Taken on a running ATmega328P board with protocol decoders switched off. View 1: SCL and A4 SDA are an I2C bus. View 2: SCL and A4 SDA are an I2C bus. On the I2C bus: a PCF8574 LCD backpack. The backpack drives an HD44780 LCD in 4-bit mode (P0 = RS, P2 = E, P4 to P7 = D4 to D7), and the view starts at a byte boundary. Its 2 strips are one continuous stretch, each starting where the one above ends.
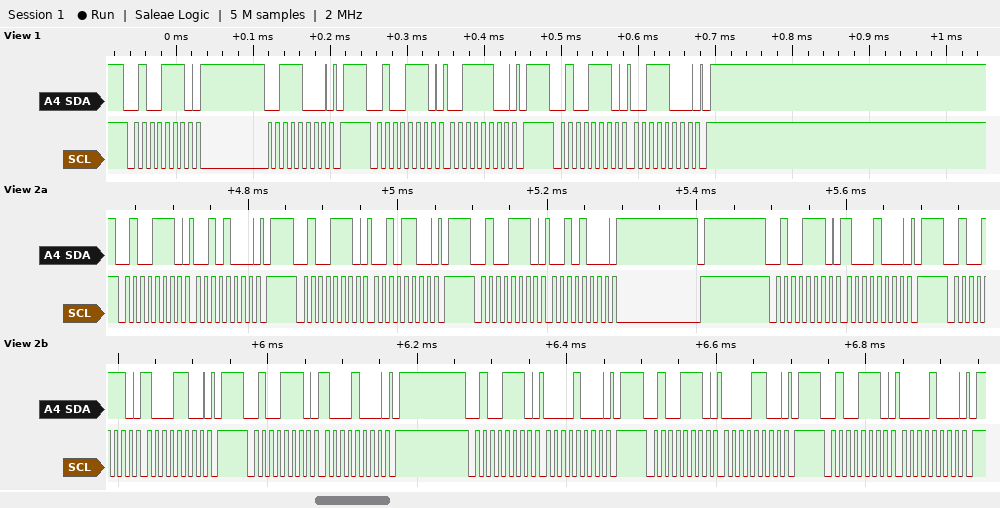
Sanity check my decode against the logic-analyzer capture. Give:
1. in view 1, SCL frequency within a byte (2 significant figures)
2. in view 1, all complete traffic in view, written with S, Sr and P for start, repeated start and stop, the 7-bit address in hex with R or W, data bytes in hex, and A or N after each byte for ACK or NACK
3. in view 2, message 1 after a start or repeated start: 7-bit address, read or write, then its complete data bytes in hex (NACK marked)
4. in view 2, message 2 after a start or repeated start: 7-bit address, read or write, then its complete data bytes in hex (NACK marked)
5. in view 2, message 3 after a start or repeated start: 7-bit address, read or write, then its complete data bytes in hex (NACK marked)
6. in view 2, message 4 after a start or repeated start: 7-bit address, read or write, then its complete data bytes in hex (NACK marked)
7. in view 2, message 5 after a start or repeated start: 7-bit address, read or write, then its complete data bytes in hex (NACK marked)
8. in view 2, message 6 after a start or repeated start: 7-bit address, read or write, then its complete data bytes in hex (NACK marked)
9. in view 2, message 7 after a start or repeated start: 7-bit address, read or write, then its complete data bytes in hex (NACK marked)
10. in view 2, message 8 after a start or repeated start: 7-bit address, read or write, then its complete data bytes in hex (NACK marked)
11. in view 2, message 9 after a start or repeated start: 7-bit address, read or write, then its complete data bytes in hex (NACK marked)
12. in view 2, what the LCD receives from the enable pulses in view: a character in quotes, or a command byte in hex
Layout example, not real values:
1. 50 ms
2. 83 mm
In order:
1. 100 kHz
2. S 27W A 38 A P S 27W A 3C A P S 27W A 38 A P
3. 0x27 write: 28
4. 0x27 write: 2C
5. 0x27 write: 28
6. 0x27 write: 88
7. 0x27 write: 8C
8. 0x27 write: 88
9. 0x27 write: 08
10. 0x27 write: 0C
11. 0x27 write: 08
12. 0x28
